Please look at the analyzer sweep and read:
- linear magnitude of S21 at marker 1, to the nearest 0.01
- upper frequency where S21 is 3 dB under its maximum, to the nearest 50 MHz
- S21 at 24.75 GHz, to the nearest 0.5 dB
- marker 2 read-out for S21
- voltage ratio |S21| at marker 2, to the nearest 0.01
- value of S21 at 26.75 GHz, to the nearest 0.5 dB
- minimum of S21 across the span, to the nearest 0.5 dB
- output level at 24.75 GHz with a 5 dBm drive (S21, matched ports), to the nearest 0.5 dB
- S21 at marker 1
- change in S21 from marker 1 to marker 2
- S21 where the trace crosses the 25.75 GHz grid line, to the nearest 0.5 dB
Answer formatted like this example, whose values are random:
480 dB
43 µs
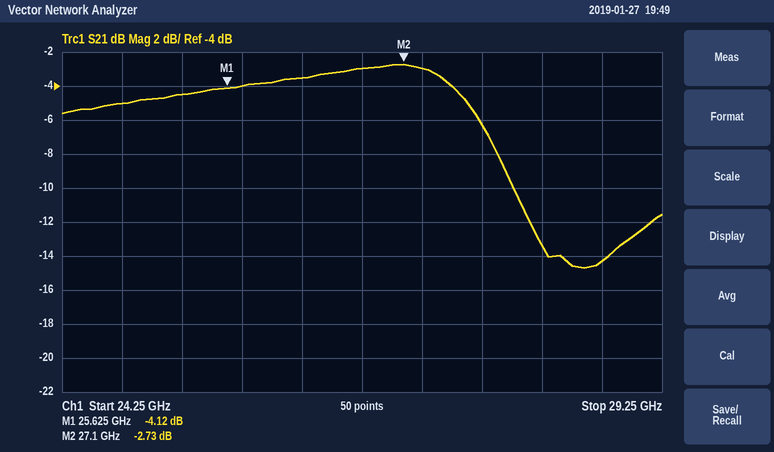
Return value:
0.62
27.70 GHz
-5.0 dB
-2.73 dB
0.73
-3.0 dB
-14.5 dB
0.0 dBm
-4.12 dB
1.39 dB
-4.0 dB
